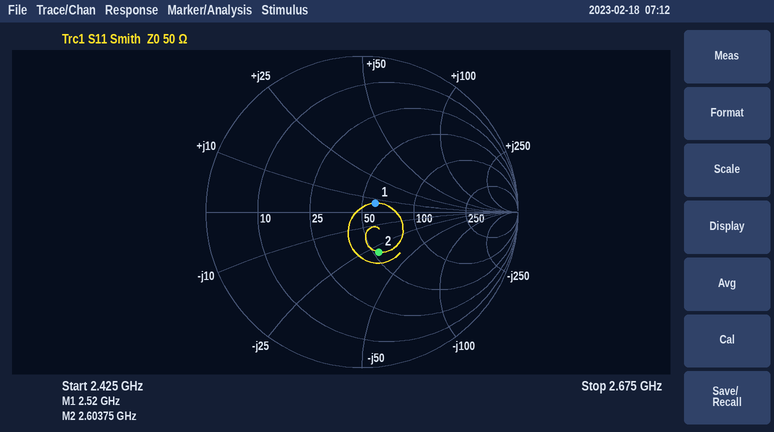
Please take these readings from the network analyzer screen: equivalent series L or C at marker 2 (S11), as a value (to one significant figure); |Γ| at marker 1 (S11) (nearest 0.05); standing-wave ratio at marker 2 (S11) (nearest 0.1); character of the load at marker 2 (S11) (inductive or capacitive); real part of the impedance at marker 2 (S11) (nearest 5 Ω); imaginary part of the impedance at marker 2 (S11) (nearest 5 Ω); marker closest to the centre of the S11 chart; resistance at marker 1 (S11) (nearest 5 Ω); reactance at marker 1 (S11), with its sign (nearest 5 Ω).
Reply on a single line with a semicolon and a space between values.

2 pF; 0.10; 1.8; capacitive; 55 Ω; -30 Ω; marker 1; 60 Ω; +5 Ω
